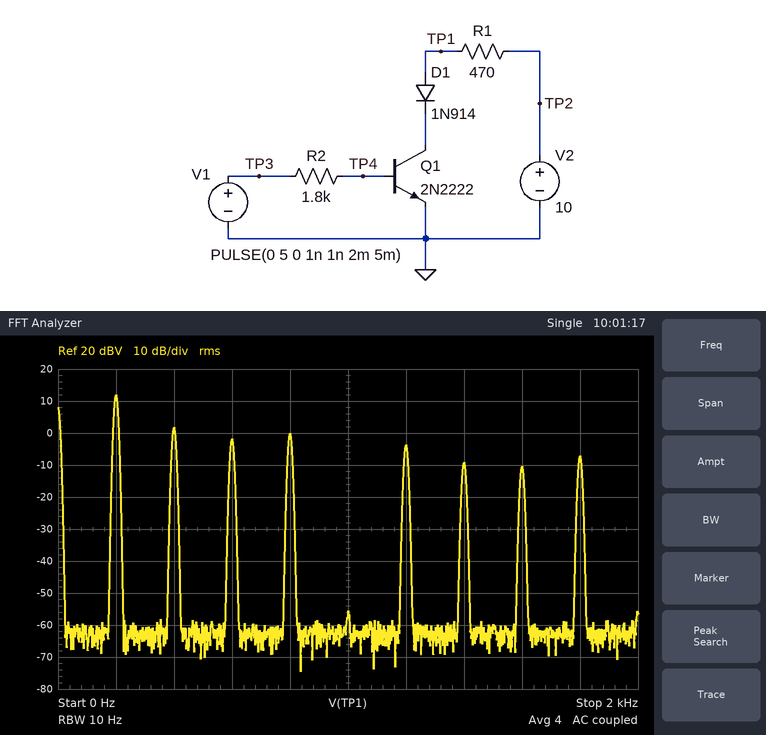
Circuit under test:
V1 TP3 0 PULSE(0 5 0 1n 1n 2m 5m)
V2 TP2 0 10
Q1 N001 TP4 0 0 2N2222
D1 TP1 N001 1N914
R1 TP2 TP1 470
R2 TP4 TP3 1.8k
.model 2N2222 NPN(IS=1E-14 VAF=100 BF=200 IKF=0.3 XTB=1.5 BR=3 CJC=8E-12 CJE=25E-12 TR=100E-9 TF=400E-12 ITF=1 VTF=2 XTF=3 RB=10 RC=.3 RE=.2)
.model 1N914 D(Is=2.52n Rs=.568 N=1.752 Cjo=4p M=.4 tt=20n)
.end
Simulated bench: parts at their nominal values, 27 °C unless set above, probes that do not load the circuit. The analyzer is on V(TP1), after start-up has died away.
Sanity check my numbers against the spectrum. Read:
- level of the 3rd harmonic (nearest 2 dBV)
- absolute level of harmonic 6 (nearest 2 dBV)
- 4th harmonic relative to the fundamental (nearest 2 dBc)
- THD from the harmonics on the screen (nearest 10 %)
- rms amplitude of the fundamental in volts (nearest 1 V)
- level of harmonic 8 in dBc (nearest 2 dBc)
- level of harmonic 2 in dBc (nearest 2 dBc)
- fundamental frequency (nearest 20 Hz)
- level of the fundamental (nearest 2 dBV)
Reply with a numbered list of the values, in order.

1. -2 dBV
2. -4 dBV
3. -12 dBc
4. 50 %
5. 4 V
6. -22 dBc
7. -10 dBc
8. 200 Hz
9. 12 dBV
